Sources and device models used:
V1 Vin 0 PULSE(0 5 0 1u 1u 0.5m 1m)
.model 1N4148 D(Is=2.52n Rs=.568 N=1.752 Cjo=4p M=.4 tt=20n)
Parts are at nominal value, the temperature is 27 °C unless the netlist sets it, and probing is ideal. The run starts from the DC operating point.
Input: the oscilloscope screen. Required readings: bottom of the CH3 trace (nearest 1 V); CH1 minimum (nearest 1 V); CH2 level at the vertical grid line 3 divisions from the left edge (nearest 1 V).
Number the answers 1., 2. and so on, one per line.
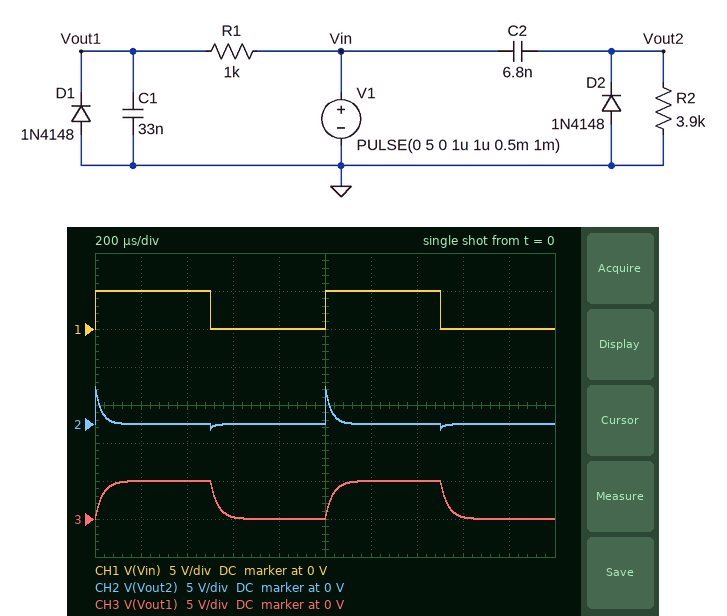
1. 0 V
2. 0 V
3. 0 V
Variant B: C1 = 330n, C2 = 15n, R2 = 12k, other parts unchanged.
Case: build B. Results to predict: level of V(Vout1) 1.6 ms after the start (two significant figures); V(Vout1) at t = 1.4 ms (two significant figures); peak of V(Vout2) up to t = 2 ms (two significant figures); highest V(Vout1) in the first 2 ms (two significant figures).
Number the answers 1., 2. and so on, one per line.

1. 3.0 V
2. 3.8 V
3. 5.0 V
4. 4.1 V
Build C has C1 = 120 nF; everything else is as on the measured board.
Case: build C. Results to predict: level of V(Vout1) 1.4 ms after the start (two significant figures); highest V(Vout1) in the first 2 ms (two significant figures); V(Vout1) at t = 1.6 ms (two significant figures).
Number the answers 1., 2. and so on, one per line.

1. 4.8 V
2. 4.9 V
3. 2.2 V
